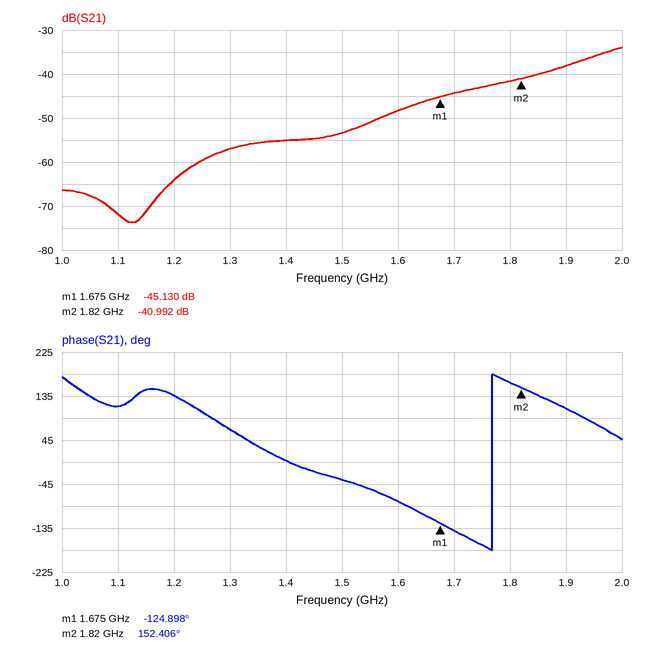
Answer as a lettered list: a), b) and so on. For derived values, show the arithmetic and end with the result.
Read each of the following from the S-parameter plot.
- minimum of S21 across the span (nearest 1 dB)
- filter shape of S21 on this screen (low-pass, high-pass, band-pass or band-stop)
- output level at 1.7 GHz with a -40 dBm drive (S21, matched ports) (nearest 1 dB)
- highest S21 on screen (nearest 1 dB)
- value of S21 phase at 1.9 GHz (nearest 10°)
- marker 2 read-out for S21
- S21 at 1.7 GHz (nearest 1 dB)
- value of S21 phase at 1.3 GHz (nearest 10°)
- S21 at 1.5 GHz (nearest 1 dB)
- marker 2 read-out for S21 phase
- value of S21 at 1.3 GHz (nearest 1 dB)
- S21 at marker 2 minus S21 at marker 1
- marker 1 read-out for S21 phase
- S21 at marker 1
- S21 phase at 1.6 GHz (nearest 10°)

a) -74 dB
b) high-pass
c) -40 dBm + (-44 dB) = -84 dBm
d) -34 dB
e) 110°
f) -40.992 dB
g) -44 dB
h) 70°
i) -53 dB
j) 152.406°
k) -57 dB
l) -40.992 − (-45.13) = 4.138 dB
m) -124.898°
n) -45.130 dB
o) -80°
